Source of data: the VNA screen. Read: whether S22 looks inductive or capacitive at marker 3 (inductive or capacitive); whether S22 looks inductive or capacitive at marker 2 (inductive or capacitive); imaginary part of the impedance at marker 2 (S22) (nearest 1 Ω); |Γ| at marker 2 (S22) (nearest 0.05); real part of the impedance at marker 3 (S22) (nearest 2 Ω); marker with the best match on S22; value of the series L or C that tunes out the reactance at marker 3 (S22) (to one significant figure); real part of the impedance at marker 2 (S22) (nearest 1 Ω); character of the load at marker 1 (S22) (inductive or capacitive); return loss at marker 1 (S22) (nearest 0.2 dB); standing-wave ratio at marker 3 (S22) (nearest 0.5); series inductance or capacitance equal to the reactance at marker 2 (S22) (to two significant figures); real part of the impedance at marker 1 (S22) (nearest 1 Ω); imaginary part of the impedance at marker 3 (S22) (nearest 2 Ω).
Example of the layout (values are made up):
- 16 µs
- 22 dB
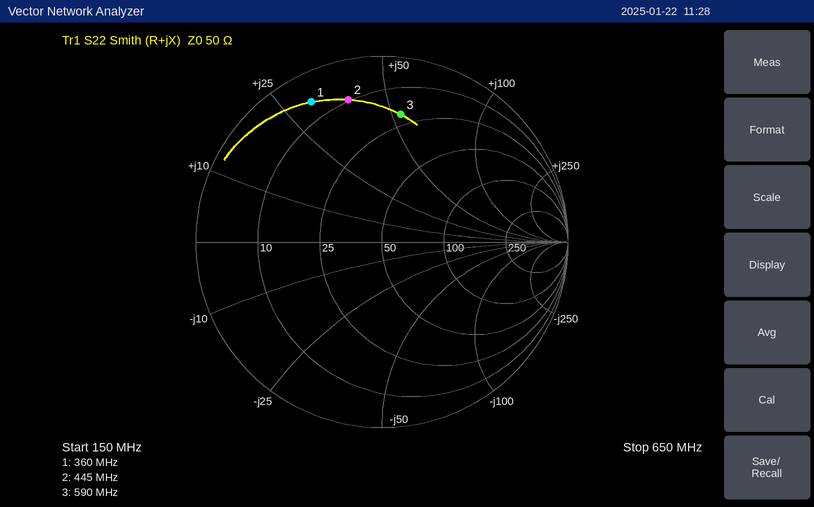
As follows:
- inductive
- inductive
- +39 Ω
- 0.80
- 20 Ω
- marker 3
- 5 pF
- 10 Ω
- inductive
- 1.4 dB
- 5.5
- 14 nH
- 6 Ω
- +54 Ω
